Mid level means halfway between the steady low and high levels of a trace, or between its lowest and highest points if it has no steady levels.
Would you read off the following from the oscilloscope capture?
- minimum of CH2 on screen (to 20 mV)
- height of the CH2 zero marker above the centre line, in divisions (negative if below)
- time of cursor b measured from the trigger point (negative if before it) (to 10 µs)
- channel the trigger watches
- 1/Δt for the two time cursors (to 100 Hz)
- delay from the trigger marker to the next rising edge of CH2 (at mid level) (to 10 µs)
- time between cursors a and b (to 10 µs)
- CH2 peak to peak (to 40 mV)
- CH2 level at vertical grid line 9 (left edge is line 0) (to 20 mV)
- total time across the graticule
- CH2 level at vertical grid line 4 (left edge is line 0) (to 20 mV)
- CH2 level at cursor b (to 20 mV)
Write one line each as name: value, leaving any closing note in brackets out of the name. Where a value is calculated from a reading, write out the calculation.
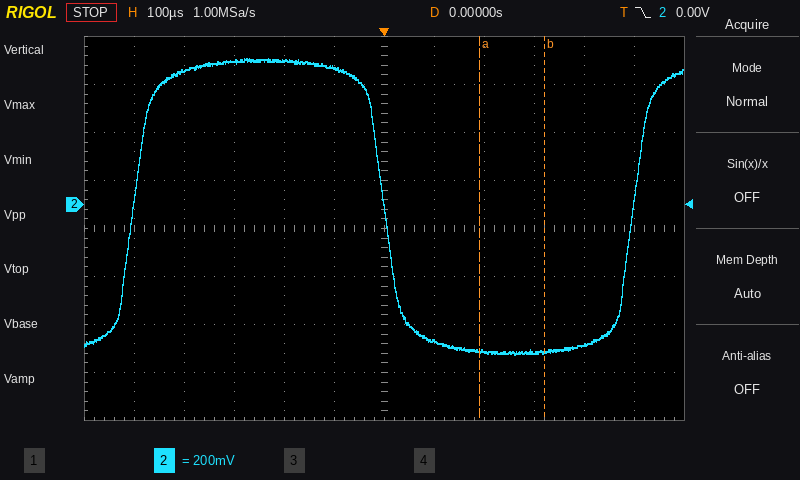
minimum of CH2 on screen: -620 mV
height of the CH2 zero marker above the centre line, in divisions: +0.5 div
time of cursor b measured from the trigger point (negative if before it): +320 µs
channel the trigger watches: CH2
1/Δt for the two time cursors: 1 / 130 µs ≈ 7.7 kHz
delay from the trigger marker to the next rising edge of CH2 (at mid level): 500 µs
time between cursors a and b: 130 µs
CH2 peak to peak: 1.24 V
CH2 level at vertical grid line 9 (left edge is line 0): -620 mV
total time across the graticule: 1.2 ms
CH2 level at vertical grid line 4 (left edge is line 0): 600 mV
CH2 level at cursor b: -620 mV
